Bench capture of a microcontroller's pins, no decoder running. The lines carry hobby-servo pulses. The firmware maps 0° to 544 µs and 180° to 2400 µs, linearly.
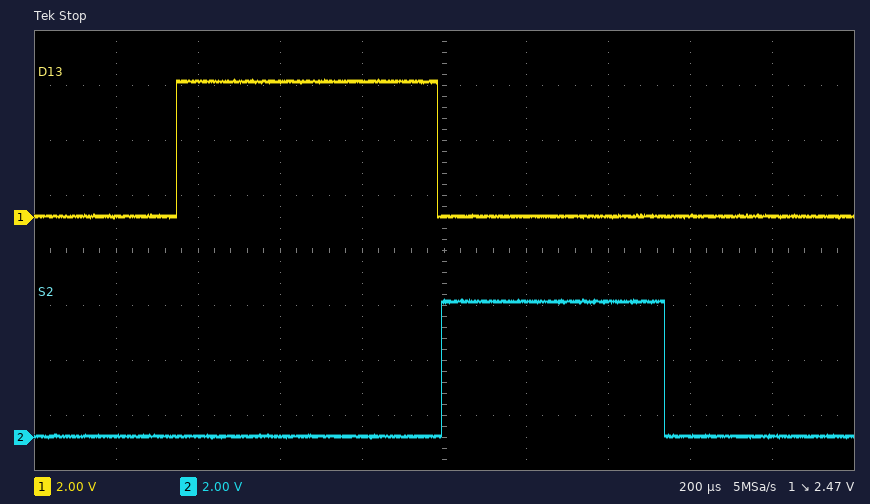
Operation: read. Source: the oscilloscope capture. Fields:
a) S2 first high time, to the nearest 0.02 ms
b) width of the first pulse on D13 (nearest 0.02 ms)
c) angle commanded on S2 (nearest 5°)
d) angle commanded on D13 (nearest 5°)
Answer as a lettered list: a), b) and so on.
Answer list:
a) 0.54 ms
b) 0.64 ms
c) 0°
d) 10°
